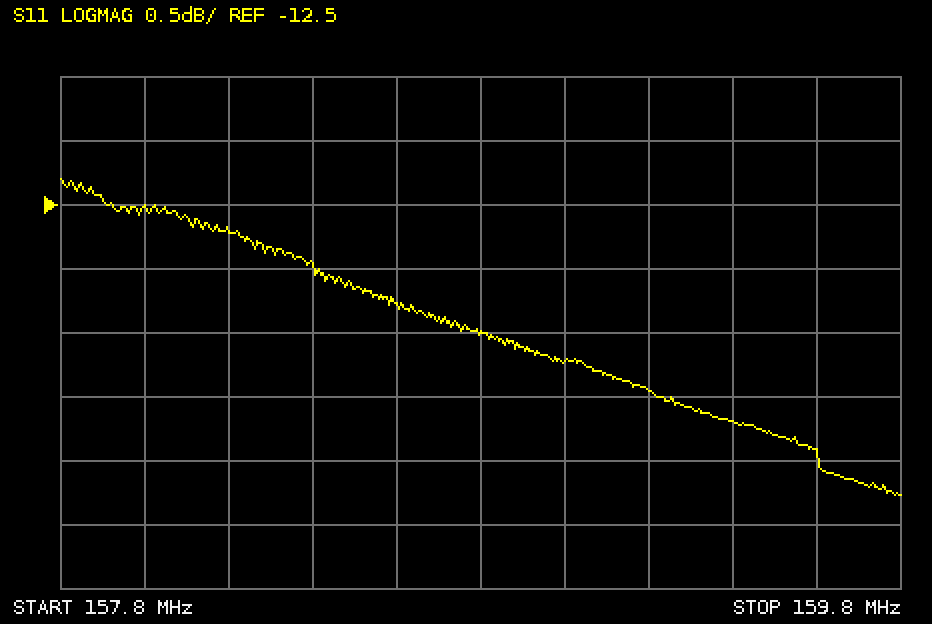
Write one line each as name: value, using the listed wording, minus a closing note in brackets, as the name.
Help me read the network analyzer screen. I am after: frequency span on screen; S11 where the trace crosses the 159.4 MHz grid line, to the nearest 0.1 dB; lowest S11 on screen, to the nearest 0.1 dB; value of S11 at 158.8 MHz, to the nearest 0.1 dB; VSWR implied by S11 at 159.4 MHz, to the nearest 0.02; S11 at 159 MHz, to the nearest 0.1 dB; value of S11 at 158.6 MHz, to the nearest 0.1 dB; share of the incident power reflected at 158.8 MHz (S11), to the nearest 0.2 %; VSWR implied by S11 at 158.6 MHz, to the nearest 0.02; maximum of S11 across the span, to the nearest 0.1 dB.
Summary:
frequency span on screen: 2 MHz
S11 where the trace crosses the 159.4 MHz grid line, to the nearest 0.1 dB: -14.2 dB
lowest S11 on screen, to the nearest 0.1 dB: -14.8 dB
value of S11 at 158.8 MHz, to the nearest 0.1 dB: -13.5 dB
VSWR implied by S11 at 159.4 MHz, to the nearest 0.02: 1.48
S11 at 159 MHz, to the nearest 0.1 dB: -13.7 dB
value of S11 at 158.6 MHz, to the nearest 0.1 dB: -13.3 dB
share of the incident power reflected at 158.8 MHz (S11), to the nearest 0.2 %: 4.4 %
VSWR implied by S11 at 158.6 MHz, to the nearest 0.02: 1.56
maximum of S11 across the span, to the nearest 0.1 dB: -12.3 dB
